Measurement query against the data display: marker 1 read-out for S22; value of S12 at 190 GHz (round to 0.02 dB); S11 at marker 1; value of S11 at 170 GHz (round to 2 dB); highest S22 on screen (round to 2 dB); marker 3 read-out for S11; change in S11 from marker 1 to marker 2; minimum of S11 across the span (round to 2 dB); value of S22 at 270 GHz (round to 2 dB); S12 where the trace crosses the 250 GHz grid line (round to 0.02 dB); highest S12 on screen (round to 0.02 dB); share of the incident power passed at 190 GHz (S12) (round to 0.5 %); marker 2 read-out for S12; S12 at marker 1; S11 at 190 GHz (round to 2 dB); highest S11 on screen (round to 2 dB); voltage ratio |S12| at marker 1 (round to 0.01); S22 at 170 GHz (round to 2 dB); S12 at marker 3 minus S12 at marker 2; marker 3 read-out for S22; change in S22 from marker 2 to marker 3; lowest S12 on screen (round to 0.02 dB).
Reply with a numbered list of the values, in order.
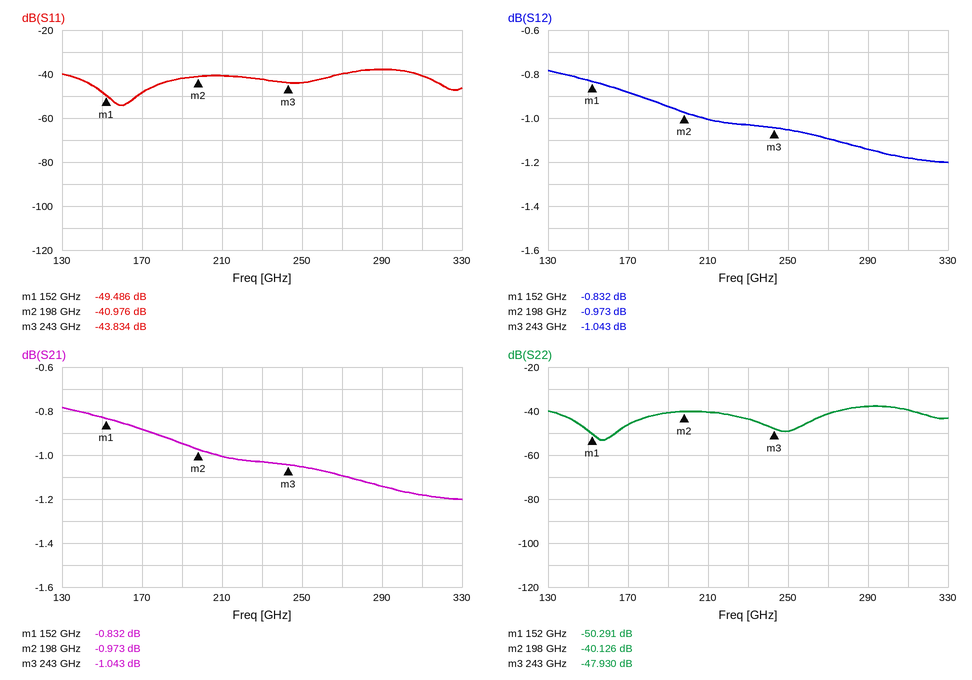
1. -50.291 dB
2. -0.94 dB
3. -49.486 dB
4. -48 dB
5. -38 dB
6. -43.834 dB
7. 8.510 dB
8. -54 dB
9. -42 dB
10. -1.06 dB
11. -0.78 dB
12. 80.5 %
13. -0.973 dB
14. -0.832 dB
15. -42 dB
16. -38 dB
17. 0.91
18. -46 dB
19. -0.070 dB
20. -47.930 dB
21. -7.804 dB
22. -1.20 dB
